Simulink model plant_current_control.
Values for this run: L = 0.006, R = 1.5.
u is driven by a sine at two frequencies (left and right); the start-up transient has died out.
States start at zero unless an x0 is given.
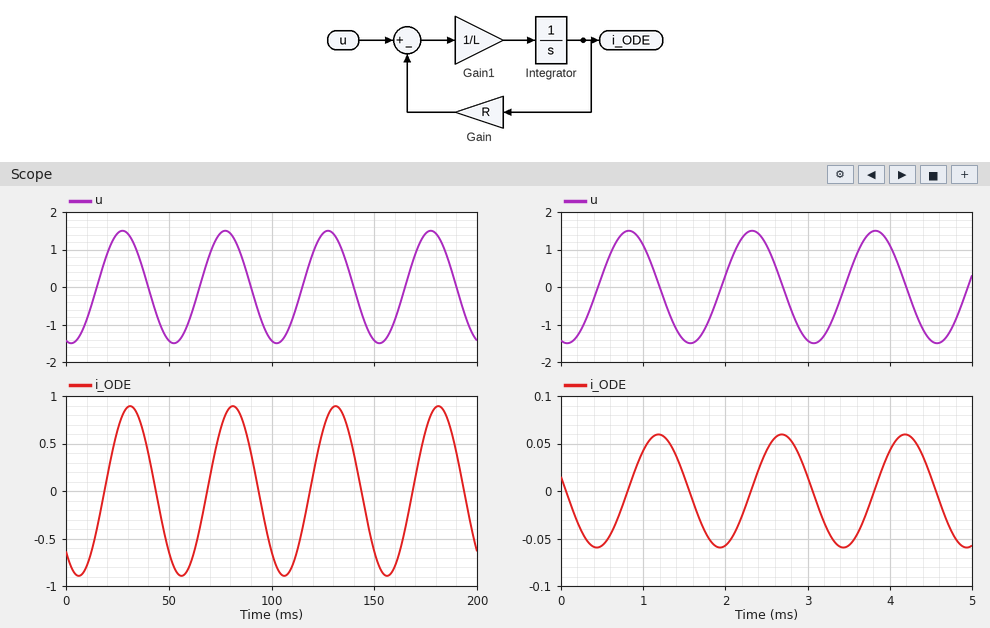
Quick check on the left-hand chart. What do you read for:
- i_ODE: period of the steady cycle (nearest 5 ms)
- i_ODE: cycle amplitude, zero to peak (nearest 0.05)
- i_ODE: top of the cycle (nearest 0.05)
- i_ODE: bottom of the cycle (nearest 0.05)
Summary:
50 ms
0.90
0.90
-0.90
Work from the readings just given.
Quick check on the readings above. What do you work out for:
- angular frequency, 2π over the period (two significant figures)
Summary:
0.13 rad/ms
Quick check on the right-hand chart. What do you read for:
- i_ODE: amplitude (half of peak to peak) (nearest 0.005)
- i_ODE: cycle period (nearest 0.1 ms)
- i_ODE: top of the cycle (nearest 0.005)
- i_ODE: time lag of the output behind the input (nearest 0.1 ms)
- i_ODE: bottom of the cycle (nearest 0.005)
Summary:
0.060
1.5 ms
0.060
0.4 ms
-0.060
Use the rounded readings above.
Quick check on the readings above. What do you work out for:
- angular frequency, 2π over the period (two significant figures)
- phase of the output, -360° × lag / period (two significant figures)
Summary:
4.2 rad/ms
-96°
